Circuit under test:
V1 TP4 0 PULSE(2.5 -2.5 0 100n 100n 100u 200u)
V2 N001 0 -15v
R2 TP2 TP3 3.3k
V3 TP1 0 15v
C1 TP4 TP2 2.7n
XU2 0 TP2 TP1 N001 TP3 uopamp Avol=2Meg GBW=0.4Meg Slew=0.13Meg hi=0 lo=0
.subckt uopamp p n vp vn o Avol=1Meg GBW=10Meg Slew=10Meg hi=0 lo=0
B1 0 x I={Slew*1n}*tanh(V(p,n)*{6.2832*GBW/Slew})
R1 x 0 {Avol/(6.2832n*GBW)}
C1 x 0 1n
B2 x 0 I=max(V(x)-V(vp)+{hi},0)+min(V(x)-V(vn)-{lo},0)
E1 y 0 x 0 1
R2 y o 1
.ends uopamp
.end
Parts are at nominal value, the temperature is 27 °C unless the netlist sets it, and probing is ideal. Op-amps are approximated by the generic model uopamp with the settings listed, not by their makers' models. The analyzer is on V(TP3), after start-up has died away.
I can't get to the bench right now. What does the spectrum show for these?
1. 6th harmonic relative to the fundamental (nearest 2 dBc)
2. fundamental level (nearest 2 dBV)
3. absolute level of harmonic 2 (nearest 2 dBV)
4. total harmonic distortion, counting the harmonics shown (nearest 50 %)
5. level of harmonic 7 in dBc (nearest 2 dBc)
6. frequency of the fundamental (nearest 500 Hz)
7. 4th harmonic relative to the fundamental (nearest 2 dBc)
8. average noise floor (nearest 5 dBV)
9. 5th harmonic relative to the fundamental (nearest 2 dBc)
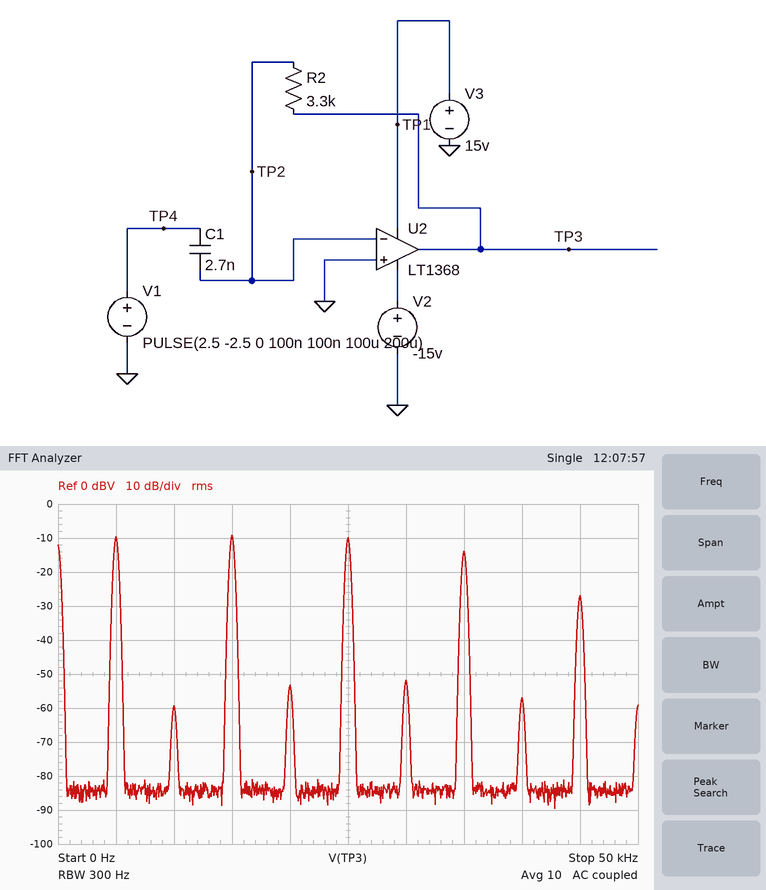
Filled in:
-42 dBc
-10 dBV
-60 dBV
150 %
-4 dBc
5.0 kHz
-44 dBc
-85 dBV
0 dBc
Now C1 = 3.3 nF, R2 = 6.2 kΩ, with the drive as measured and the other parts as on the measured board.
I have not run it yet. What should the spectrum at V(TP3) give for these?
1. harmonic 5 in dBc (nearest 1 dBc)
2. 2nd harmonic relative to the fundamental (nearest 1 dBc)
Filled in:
-17 dBc
-47 dBc
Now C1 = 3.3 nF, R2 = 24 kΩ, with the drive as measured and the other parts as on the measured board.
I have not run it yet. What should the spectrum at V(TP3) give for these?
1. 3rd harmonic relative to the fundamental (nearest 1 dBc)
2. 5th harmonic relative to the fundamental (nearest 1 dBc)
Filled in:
-19 dBc
-28 dBc
